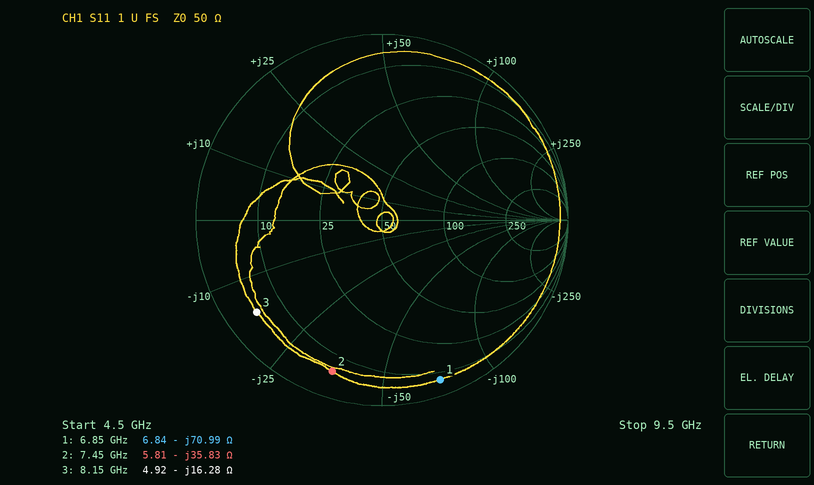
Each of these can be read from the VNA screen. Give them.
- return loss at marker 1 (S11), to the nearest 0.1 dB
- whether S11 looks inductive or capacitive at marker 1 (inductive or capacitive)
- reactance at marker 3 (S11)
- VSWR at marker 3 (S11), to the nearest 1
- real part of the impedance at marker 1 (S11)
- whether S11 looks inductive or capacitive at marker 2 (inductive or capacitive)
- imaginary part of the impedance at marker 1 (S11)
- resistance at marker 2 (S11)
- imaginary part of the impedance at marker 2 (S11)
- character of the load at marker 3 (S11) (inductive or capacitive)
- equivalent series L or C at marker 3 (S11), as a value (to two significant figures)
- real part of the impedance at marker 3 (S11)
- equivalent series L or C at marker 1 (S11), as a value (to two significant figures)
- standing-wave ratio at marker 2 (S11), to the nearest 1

0.8 dB
capacitive
-16.28 Ω
11
6.84 Ω
capacitive
-70.99 Ω
5.81 Ω
-35.83 Ω
capacitive
1.2 pF
4.92 Ω
330 fF
13
